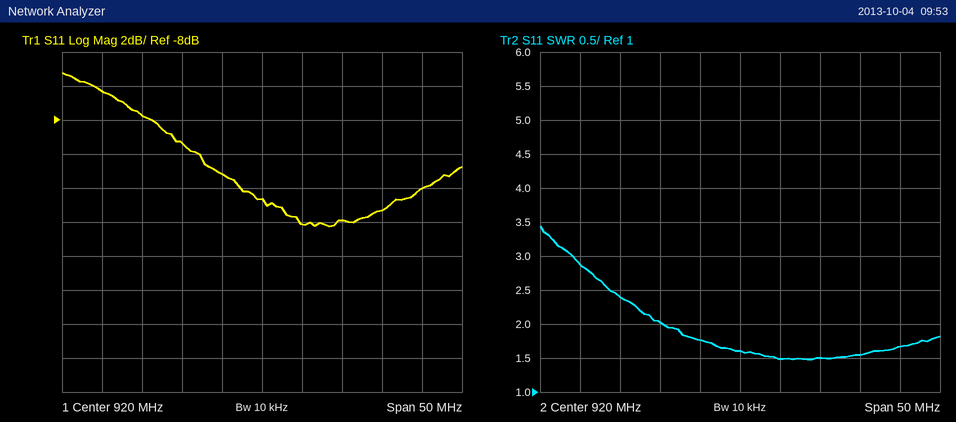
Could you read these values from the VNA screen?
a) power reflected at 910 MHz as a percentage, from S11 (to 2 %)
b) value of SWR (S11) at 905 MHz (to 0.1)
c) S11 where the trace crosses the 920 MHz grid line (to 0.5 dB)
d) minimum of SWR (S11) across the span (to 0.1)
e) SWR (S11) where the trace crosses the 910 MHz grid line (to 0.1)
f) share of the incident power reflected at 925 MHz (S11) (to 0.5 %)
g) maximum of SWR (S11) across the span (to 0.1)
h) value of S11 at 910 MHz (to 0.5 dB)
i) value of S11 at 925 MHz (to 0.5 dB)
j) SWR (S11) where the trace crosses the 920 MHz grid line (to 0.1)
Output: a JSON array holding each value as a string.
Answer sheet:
["12 %", "2.4", "-12.5 dB", "1.5", "2.0", "4.0 %", "3.4", "-9.5 dB", "-14.0 dB", "1.6"]
